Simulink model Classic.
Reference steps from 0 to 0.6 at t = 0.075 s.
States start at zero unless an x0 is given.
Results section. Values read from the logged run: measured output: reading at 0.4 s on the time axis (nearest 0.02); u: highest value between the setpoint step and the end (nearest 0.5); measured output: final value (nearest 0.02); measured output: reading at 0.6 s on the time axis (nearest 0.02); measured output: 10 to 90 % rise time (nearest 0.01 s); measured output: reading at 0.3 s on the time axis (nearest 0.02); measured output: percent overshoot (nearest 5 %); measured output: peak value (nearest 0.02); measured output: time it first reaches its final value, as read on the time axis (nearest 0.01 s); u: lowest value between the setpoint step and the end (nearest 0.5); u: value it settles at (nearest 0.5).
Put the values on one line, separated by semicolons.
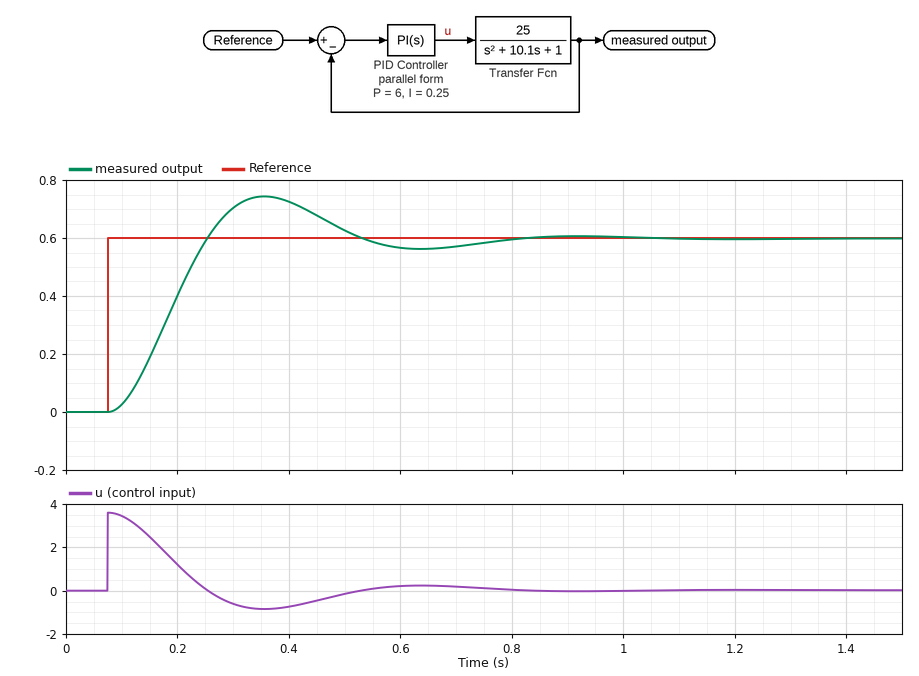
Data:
0.72; 3.5; 0.60; 0.56; 0.12 s; 0.70; 25 %; 0.74; 0.25 s; -1.0; 0.0
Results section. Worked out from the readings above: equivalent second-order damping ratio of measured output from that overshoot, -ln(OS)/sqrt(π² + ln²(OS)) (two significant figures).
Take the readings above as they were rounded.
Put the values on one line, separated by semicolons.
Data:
0.40
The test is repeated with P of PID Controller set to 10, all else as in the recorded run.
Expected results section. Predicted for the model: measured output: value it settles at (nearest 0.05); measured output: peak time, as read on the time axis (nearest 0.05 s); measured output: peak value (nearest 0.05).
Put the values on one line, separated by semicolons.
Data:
0.60; 0.30 s; 0.80
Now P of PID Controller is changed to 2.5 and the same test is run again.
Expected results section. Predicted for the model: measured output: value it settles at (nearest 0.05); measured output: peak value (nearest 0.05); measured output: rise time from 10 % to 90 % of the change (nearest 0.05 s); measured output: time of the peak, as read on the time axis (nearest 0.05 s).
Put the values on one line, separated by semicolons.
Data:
0.60; 0.65; 0.25 s; 0.60 s
